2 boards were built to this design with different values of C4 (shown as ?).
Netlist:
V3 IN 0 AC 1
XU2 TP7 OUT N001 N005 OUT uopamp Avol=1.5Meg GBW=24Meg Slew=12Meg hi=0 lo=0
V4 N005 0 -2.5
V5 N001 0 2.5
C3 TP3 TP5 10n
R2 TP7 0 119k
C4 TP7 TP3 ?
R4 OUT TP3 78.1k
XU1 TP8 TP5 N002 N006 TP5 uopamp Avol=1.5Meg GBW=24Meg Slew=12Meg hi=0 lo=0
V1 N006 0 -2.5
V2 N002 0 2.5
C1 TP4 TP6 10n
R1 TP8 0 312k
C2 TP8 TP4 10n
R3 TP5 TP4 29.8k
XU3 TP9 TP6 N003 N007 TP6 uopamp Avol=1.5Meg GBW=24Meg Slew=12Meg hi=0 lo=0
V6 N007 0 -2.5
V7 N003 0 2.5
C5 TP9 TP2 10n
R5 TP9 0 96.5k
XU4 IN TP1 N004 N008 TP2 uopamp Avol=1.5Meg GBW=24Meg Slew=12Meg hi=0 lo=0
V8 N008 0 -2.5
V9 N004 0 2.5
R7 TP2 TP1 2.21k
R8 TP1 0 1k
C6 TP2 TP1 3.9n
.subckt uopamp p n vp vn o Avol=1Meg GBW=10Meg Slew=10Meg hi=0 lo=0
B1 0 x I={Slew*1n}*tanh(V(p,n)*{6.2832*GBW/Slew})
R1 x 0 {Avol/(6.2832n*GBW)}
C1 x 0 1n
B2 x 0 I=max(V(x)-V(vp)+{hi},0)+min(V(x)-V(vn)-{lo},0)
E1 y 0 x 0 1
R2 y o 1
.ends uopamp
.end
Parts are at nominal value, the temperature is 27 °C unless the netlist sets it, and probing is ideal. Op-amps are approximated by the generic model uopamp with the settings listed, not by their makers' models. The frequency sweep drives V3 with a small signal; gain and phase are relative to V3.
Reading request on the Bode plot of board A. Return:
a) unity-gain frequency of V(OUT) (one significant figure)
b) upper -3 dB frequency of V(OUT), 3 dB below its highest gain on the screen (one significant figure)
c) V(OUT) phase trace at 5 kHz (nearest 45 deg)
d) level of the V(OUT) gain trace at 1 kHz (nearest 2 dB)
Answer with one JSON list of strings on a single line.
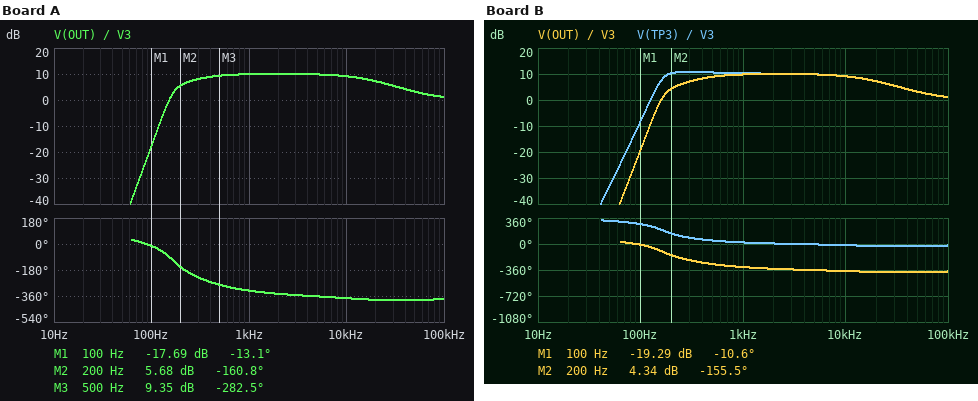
["200 Hz", "20 kHz", "-360 deg", "10 dB"]
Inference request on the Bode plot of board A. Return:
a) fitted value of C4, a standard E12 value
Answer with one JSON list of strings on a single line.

["4.7 nF"]
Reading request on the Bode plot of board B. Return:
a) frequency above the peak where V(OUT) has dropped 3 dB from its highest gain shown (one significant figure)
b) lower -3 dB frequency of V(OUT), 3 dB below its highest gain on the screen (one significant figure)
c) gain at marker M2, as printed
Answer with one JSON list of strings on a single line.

["20 kHz", "300 Hz", "4.34 dB"]
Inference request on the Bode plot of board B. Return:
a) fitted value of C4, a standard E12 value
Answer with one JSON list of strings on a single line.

["3.9 nF"]
